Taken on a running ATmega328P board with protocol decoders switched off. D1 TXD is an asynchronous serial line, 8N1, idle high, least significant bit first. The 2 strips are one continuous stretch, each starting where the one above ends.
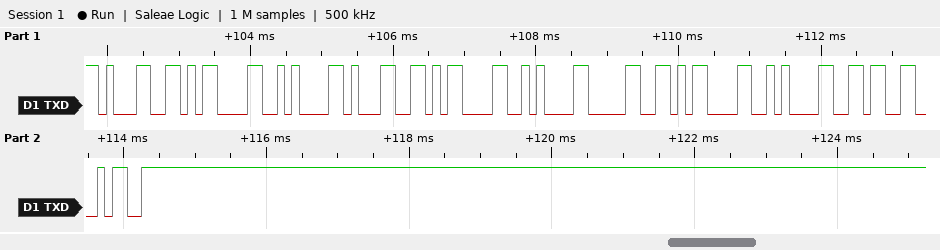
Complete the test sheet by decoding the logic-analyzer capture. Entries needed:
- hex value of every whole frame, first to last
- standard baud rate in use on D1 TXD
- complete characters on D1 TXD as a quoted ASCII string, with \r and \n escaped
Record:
0x31 0x0D 0x0A 0x31 0x0D 0x0A 0x30 0x0D 0x0A 0x36 0x34
9600 baud
"1\r\n1\r\n0\r\n64"
